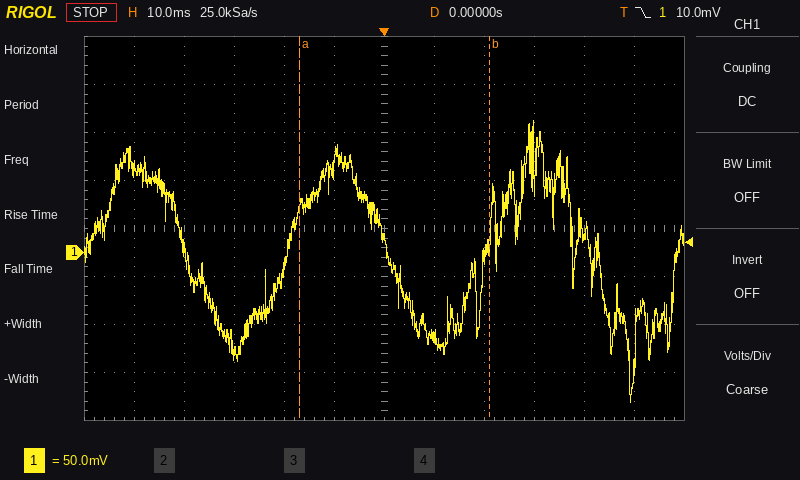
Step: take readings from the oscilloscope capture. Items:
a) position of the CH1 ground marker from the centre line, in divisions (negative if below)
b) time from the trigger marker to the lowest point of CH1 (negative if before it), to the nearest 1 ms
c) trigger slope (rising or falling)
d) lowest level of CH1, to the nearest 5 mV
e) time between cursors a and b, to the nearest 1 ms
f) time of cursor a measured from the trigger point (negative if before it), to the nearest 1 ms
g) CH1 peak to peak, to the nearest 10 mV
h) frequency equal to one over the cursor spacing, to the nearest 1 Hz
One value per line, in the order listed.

-0.5 div
+49 ms
falling
-155 mV
38 ms
-17 ms
290 mV
26 Hz
